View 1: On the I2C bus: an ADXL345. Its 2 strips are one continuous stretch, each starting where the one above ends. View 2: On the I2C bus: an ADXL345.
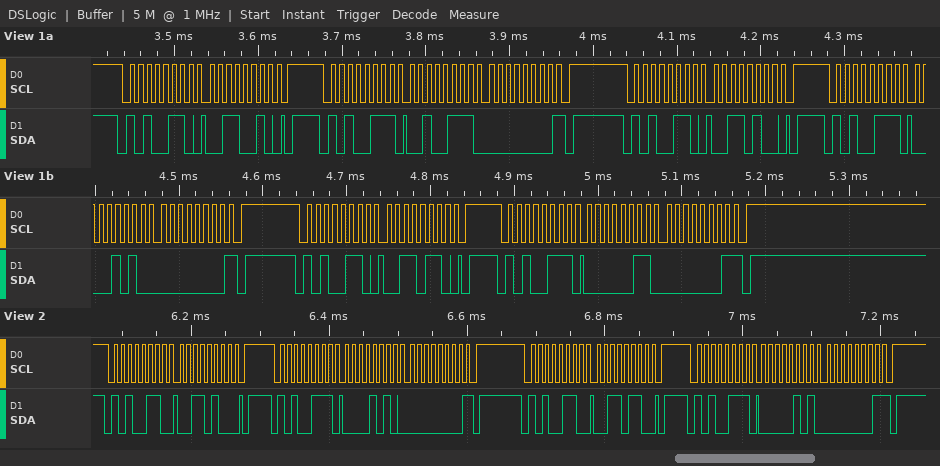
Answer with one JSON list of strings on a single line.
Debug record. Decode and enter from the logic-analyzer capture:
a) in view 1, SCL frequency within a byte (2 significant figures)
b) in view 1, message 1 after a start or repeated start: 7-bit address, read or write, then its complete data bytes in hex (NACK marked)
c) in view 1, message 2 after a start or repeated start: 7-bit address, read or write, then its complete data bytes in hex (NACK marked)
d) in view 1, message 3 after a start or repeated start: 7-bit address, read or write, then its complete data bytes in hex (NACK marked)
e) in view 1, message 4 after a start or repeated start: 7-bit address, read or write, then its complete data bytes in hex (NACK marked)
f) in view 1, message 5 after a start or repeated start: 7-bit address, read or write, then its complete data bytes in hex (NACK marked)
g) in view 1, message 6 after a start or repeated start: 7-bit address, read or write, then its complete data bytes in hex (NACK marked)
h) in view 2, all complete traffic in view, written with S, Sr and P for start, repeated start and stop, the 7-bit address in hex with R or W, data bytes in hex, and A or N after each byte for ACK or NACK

["100 kHz", "0x53 write: 32", "0x53 read: 27 00 NACK", "0x53 write: 34", "0x53 read: 0A 00 NACK", "0x53 write: 36", "0x53 read: 03 01 NACK", "S 53W A 34 A P S 53R A 0A A 00 N P S 53W A 36 A P S 53R A 05 A 01 N P"]
